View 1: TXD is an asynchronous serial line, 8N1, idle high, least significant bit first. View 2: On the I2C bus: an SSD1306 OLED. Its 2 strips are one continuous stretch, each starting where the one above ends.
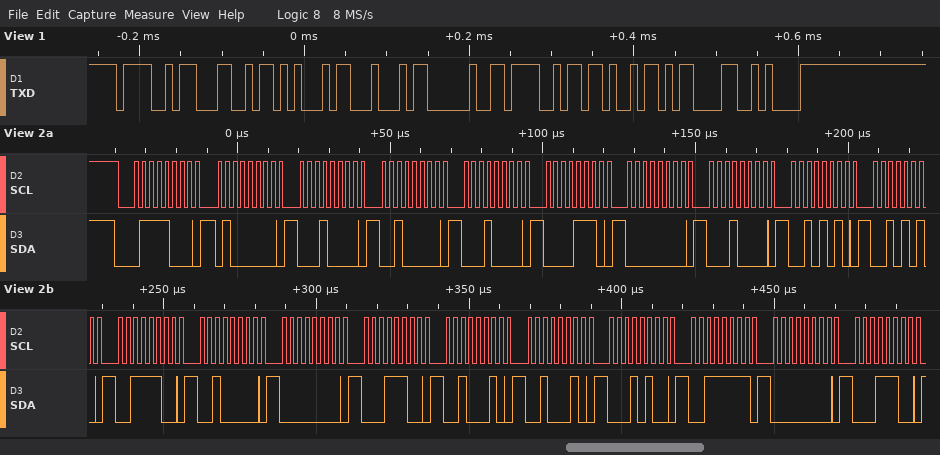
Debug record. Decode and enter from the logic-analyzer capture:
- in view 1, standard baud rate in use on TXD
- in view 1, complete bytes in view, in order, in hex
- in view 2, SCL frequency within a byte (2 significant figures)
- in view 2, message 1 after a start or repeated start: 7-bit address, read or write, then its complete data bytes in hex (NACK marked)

115200 baud
4F 4C 45 44 20 4F 4B 0D 0A
400 kHz
0x3C write: 40 10 20 10 0E 00 10 2A 2A 3C 20 00 1C 22 22 14 3F 00 1C
